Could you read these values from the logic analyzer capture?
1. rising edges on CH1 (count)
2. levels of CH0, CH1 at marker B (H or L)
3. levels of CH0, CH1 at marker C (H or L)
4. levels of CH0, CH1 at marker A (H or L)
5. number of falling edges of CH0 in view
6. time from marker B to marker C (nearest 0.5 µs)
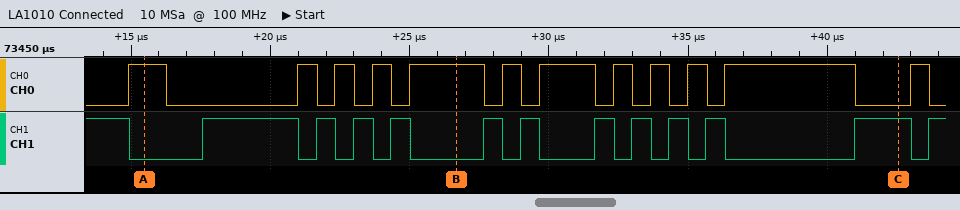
12
CH0=H, CH1=L
CH0=L, CH1=H
CH0=H, CH1=L
12
16 µs
